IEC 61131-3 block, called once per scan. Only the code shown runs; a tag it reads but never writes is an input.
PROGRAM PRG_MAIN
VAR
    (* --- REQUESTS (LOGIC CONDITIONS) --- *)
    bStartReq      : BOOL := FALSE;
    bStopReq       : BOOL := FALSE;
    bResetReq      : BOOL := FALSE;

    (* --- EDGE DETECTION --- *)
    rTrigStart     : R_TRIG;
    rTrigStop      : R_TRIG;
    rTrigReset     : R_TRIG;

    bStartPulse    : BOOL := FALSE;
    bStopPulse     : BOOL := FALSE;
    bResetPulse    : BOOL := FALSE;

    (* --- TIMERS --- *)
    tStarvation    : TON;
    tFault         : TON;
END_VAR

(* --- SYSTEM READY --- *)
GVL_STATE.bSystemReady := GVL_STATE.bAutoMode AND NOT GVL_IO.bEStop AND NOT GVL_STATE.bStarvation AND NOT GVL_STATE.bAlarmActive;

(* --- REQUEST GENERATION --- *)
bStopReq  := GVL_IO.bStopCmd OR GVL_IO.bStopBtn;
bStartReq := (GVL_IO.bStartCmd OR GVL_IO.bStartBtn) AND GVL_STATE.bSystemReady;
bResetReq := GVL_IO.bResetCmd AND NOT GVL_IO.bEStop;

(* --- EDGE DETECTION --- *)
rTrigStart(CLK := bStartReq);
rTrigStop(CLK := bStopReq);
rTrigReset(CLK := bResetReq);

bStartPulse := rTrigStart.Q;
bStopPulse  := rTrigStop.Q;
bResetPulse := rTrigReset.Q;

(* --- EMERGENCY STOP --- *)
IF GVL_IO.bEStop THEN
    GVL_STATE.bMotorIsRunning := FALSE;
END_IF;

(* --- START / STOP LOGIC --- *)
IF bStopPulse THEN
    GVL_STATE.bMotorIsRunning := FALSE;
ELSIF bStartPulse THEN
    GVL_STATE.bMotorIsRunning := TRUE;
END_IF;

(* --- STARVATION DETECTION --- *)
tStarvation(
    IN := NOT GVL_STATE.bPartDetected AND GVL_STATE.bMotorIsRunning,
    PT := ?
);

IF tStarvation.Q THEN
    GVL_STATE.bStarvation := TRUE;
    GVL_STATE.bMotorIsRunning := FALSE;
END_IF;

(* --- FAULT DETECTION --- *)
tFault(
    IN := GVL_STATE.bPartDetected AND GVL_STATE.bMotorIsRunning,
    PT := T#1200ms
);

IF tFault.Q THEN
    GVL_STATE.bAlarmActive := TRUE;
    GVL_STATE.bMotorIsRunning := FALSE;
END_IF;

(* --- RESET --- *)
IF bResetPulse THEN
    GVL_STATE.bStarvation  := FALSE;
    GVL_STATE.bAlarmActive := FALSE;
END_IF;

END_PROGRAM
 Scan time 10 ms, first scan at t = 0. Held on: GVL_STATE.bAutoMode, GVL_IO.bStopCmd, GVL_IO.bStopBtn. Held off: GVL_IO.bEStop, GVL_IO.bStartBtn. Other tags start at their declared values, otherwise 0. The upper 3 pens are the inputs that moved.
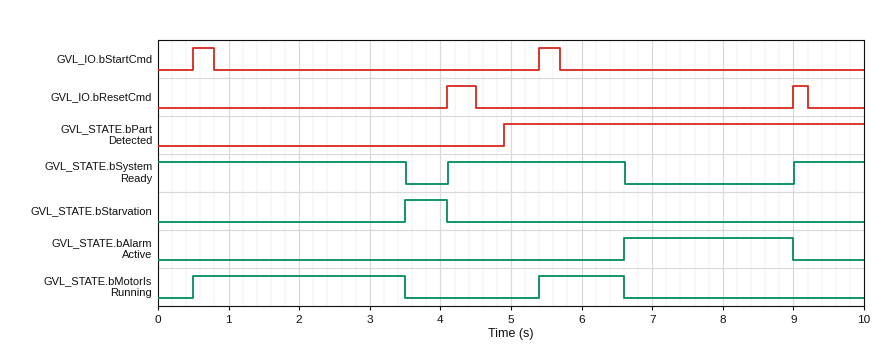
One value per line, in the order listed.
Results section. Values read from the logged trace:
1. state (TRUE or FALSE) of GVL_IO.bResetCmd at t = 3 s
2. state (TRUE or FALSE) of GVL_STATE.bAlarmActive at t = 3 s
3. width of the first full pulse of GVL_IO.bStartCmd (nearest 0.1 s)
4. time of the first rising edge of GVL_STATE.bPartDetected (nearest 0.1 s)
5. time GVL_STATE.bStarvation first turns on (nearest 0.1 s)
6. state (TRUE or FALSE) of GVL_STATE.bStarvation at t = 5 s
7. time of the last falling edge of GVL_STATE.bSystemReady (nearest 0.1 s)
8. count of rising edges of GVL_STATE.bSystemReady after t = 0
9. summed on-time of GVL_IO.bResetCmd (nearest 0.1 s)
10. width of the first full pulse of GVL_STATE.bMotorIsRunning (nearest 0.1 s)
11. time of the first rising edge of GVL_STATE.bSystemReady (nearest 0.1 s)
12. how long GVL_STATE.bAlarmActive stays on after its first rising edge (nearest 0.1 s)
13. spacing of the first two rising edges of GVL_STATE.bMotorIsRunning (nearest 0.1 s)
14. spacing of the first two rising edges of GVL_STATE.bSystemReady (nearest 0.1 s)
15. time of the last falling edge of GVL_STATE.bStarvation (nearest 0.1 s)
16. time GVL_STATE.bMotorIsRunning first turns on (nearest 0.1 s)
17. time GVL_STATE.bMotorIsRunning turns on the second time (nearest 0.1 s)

FALSE
FALSE
0.3 s
4.9 s
3.5 s
FALSE
6.6 s
2
0.6 s
3.0 s
4.1 s
2.4 s
4.9 s
4.9 s
4.1 s
0.5 s
5.4 s
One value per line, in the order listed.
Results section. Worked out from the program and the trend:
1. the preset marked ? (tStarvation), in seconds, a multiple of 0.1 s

3.0 s
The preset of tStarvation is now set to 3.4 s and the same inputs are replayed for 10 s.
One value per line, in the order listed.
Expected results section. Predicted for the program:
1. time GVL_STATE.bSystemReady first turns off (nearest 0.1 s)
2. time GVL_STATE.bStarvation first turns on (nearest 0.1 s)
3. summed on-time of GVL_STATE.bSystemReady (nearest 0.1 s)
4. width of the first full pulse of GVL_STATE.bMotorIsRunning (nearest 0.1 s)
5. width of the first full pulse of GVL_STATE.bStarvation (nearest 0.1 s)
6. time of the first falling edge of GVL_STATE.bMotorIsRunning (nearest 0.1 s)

3.9 s
3.9 s
7.4 s
3.4 s
0.2 s
3.9 s
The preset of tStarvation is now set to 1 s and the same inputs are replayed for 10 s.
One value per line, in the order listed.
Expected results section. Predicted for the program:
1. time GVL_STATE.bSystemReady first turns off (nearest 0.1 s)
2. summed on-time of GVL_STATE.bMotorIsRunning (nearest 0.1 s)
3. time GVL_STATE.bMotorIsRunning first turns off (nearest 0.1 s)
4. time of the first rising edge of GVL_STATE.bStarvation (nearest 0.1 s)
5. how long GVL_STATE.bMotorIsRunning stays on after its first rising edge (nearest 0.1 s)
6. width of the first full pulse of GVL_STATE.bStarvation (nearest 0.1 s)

1.5 s
2.2 s
1.5 s
1.5 s
1.0 s
2.6 s
